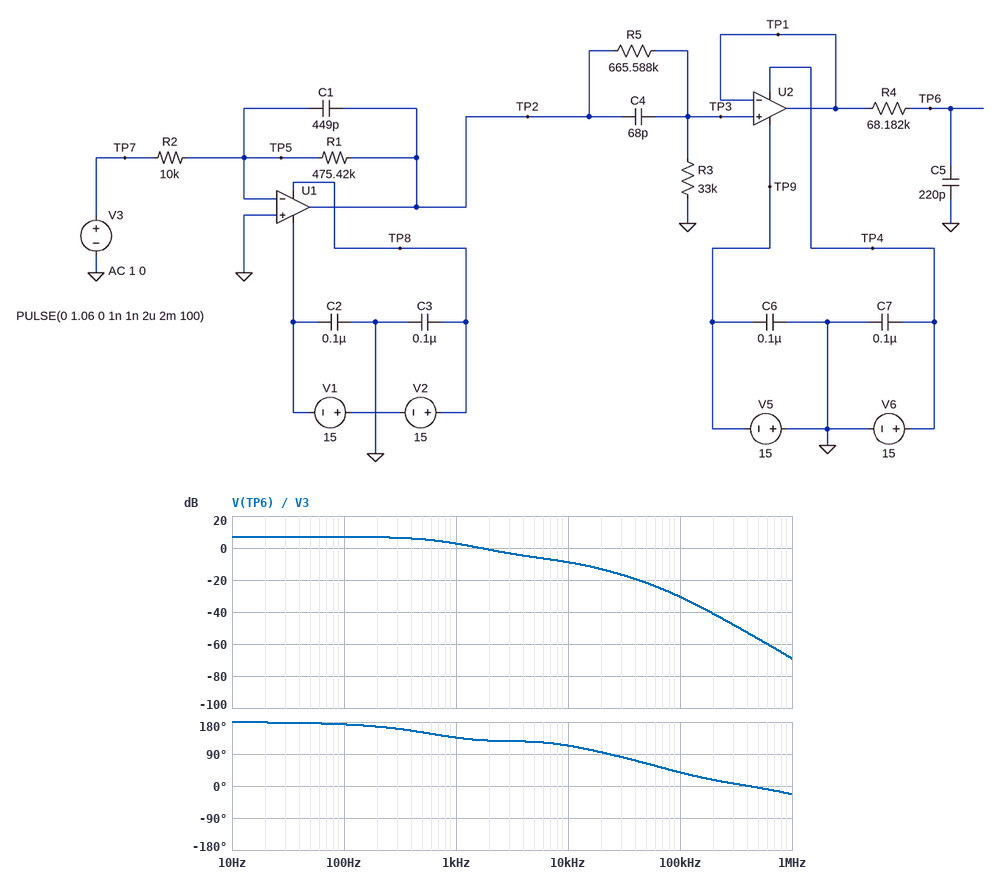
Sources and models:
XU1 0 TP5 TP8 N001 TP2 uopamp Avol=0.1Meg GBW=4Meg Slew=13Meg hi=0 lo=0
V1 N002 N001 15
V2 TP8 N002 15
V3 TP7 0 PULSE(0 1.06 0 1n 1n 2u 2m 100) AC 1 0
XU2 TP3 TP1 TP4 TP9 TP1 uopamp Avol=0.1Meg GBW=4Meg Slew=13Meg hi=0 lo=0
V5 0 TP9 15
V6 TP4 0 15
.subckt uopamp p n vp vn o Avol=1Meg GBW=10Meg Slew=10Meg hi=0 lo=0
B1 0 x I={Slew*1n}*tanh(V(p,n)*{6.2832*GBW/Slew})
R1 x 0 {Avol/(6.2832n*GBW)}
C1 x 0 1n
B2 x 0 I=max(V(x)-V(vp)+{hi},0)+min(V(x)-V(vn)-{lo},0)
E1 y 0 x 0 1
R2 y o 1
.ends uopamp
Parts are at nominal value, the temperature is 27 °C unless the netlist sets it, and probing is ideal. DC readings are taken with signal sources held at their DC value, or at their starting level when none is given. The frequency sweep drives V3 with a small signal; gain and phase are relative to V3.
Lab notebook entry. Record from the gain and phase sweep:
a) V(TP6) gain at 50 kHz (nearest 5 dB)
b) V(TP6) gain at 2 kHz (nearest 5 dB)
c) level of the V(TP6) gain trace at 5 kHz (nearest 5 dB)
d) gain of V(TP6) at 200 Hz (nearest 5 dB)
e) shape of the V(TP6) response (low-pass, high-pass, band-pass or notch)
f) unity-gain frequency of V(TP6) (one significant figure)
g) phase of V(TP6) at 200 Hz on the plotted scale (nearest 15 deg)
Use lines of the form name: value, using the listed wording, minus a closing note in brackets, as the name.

V(TP6) gain at 50 kHz: -20 dB
V(TP6) gain at 2 kHz: 0 dB
level of the V(TP6) gain trace at 5 kHz: -5 dB
gain of V(TP6) at 200 Hz: 5 dB
shape of the V(TP6) response: low-pass
unity-gain frequency of V(TP6): 2 kHz
phase of V(TP6) at 200 Hz on the plotted scale: 165 deg
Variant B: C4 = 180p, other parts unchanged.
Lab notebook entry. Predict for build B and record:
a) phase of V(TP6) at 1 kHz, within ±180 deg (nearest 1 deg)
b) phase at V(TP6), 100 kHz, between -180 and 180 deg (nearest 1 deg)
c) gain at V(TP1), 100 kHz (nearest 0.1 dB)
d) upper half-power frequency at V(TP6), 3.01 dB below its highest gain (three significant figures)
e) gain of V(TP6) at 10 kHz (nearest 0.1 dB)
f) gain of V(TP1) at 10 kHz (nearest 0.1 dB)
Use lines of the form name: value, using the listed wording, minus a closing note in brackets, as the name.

phase of V(TP6) at 1 kHz, within ±180 deg: 156 deg
phase at V(TP6), 100 kHz, between -180 and 180 deg: 19 deg
gain at V(TP1), 100 kHz: -9.4 dB
upper half-power frequency at V(TP6), 3.01 dB below its highest gain: 1.17 kHz
gain of V(TP6) at 10 kHz: -1.3 dB
gain of V(TP1) at 10 kHz: 1.5 dB
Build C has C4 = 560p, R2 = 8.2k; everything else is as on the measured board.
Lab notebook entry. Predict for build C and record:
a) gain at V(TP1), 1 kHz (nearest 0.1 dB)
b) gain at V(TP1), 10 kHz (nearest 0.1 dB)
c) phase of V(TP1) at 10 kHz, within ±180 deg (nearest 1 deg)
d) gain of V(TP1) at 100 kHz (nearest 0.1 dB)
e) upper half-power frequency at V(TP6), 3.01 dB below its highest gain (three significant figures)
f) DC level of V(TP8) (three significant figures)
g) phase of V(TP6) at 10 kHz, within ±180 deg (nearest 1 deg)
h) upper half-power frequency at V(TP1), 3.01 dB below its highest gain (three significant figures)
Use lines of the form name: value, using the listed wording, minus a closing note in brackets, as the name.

gain at V(TP1), 1 kHz: 12.3 dB
gain at V(TP1), 10 kHz: 10.0 dB
phase of V(TP1) at 10 kHz, within ±180 deg: 134 deg
gain of V(TP1) at 100 kHz: -7.4 dB
upper half-power frequency at V(TP6), 3.01 dB below its highest gain: 7.11 kHz
DC level of V(TP8): 15.0 V
phase of V(TP6) at 10 kHz, within ±180 deg: 90 deg
upper half-power frequency at V(TP1), 3.01 dB below its highest gain: 10.2 kHz
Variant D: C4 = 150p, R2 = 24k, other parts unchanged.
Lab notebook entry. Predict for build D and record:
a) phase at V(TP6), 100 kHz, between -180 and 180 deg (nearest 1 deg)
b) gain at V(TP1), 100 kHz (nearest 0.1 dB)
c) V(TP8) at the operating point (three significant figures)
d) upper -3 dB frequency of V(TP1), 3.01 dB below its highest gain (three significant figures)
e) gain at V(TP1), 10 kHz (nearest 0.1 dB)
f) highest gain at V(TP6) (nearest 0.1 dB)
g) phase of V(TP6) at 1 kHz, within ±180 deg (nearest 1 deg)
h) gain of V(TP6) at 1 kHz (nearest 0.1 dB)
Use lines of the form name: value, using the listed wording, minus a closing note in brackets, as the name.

phase at V(TP6), 100 kHz, between -180 and 180 deg: 21 deg
gain at V(TP1), 100 kHz: -17.1 dB
V(TP8) at the operating point: 15.0 V
upper -3 dB frequency of V(TP1), 3.01 dB below its highest gain: 987 Hz
gain at V(TP1), 10 kHz: -7.5 dB
highest gain at V(TP6): -0.6 dB
phase of V(TP6) at 1 kHz, within ±180 deg: 152 deg
gain of V(TP6) at 1 kHz: -3.7 dB
